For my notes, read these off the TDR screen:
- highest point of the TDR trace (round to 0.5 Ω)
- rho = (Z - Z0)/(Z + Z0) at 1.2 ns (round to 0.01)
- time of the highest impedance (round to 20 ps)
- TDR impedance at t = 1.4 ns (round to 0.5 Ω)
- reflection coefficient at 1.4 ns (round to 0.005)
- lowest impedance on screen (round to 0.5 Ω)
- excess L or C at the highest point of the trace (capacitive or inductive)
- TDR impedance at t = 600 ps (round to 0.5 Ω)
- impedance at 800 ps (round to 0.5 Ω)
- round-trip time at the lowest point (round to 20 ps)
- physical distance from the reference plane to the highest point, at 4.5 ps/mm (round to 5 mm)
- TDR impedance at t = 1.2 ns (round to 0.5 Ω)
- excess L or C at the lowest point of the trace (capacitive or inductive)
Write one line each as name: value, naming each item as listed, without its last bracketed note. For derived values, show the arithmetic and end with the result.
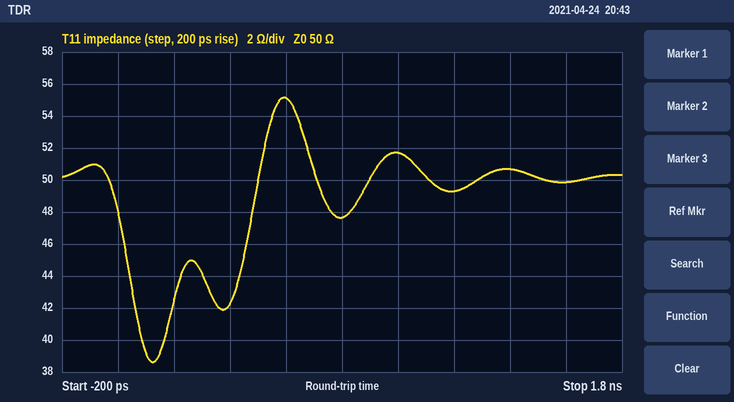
highest point of the TDR trace: 55.0 Ω
rho = (Z - Z0)/(Z + Z0) at 1.2 ns: (49.5 − 50)/(49.5 + 50) ≈ -0.01
time of the highest impedance: 600 ps
TDR impedance at t = 1.4 ns: 50.5 Ω
reflection coefficient at 1.4 ns: (50.5 − 50)/(50.5 + 50) ≈ +0.005
lowest impedance on screen: 38.5 Ω
excess L or C at the highest point of the trace: inductive
TDR impedance at t = 600 ps: 55.0 Ω
impedance at 800 ps: 47.5 Ω
round-trip time at the lowest point: 120 ps
physical distance from the reference plane to the highest point, at 4.5 ps/mm: 600 ps / 2 / 4.5 ps/mm ≈ 66.7 mm, so 65 mm to the nearest 5 mm
TDR impedance at t = 1.2 ns: 49.5 Ω
excess L or C at the lowest point of the trace: capacitive
